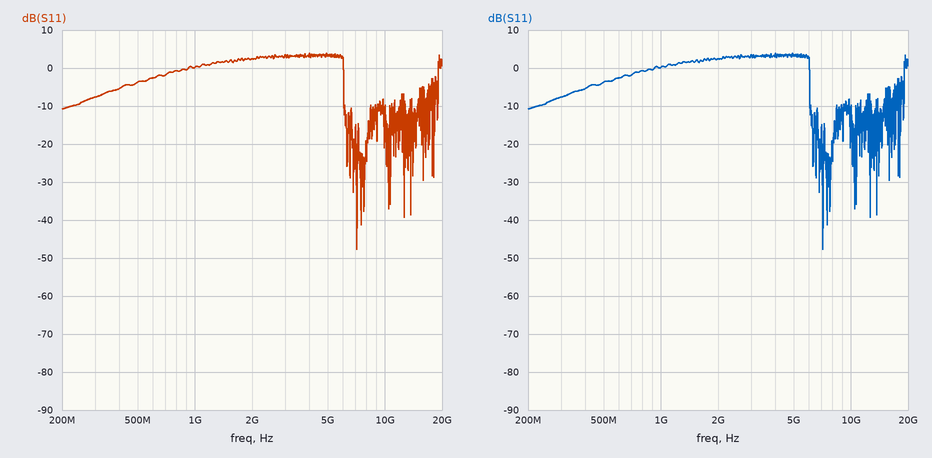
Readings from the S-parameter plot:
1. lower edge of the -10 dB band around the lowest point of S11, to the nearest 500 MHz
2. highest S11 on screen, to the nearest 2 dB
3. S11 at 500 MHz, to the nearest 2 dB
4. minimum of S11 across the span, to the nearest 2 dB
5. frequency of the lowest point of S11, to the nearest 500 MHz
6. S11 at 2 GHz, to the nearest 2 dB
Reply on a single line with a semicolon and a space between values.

6.0 GHz; 4 dB; -4 dB; -48 dB; 7.0 GHz; 2 dB
